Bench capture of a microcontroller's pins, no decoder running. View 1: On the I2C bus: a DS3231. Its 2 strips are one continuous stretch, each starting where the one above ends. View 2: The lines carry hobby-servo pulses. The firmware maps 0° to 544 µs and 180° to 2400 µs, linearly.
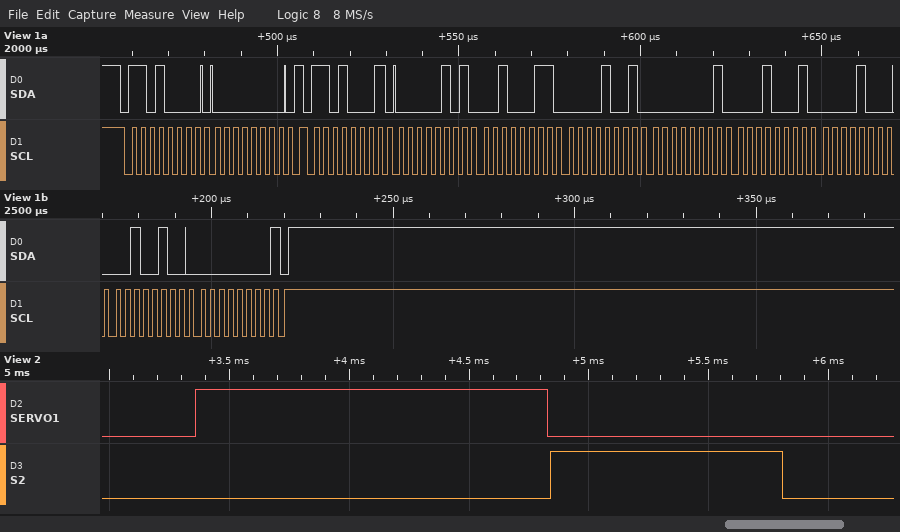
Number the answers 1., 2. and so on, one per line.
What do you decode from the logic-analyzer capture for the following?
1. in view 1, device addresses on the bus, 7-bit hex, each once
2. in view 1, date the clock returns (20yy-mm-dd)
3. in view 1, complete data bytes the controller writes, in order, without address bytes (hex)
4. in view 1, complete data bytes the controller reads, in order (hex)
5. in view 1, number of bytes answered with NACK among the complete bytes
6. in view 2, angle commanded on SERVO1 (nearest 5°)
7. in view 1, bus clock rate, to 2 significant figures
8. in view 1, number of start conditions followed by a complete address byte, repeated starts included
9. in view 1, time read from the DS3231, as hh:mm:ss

1. 0x68
2. 2024-08-11
3. 00
4. 05 23 09 01 11 08 24 00
5. 1
6. 90°
7. 400 kHz
8. 2
9. 09:23:05
